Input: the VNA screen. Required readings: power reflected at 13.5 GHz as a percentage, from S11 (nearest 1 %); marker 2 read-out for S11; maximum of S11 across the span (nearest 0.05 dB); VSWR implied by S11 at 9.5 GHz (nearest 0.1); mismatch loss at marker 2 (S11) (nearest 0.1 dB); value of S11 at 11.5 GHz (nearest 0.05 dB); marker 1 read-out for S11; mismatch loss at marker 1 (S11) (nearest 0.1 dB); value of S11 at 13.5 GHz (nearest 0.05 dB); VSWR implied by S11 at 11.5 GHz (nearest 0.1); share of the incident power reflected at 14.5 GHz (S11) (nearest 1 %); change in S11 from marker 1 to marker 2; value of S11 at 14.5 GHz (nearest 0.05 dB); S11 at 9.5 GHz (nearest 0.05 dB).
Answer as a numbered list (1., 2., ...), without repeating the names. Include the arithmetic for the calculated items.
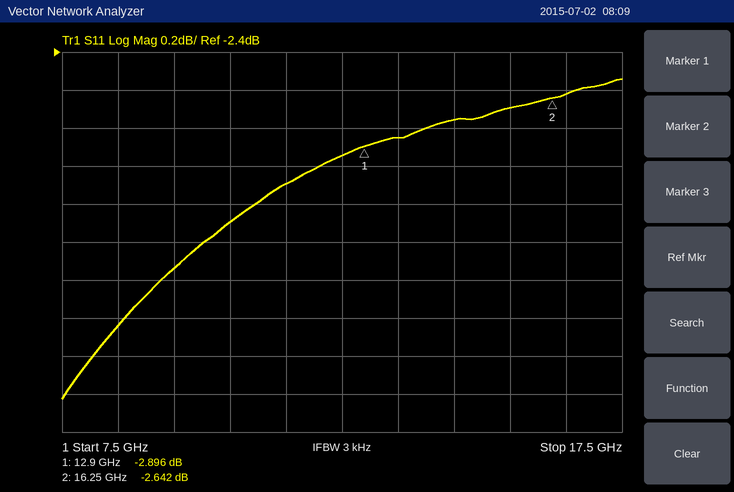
1. 10^(-2.85/10) ≈ 52 %
2. -2.642 dB
3. -2.55 dB
4. |Γ| = 10^(-3.55/20) = 0.6645; VSWR = (1 + 0.6645)/(1 − 0.6645) ≈ 5.0
5. −10 log10(1 − 10^(-2.642/10)) ≈ 3.4 dB
6. -3.10 dB
7. -2.896 dB
8. −10 log10(1 − 10^(-2.896/10)) ≈ 3.1 dB
9. -2.85 dB
10. |Γ| = 10^(-3.1/20) = 0.6998; VSWR = (1 + 0.6998)/(1 − 0.6998) ≈ 5.7
11. 10^(-2.75/10) ≈ 53 %
12. -2.642 − (-2.896) = 0.254 dB
13. -2.75 dB
14. -3.55 dB
